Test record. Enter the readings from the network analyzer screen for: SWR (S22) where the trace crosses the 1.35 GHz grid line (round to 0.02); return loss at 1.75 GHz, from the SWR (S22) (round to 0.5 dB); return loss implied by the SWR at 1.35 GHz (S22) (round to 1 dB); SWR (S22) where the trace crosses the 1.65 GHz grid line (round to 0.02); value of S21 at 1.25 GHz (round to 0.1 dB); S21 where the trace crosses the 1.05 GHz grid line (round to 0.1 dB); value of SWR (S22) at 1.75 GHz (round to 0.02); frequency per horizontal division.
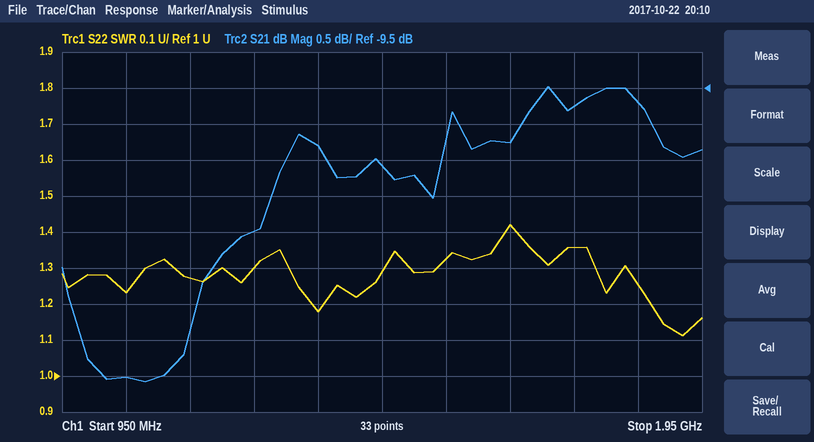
1.18
16.5 dB
22 dB
1.42
-11.5 dB
-13.5 dB
1.36
100 MHz
